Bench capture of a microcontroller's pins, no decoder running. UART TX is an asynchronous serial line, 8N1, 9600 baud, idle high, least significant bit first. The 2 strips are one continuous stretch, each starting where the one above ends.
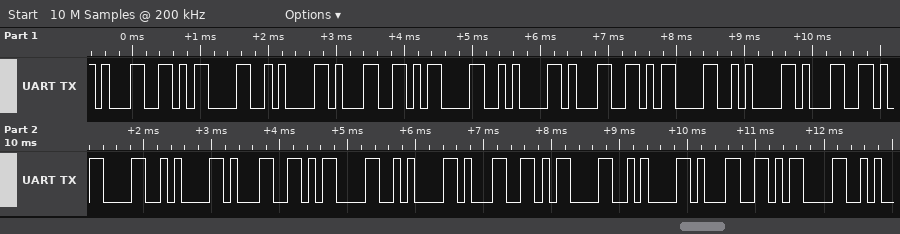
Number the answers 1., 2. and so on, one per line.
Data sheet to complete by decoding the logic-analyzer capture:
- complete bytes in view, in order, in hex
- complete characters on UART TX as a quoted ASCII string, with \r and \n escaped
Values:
1. 31 0D 0A 31 0D 0A 31 0D 0A 31 0D 0A 31 0D 0A 31 0D 0A 31 0D
2. "1\r\n1\r\n1\r\n1\r\n1\r\n1\r\n1\r"
